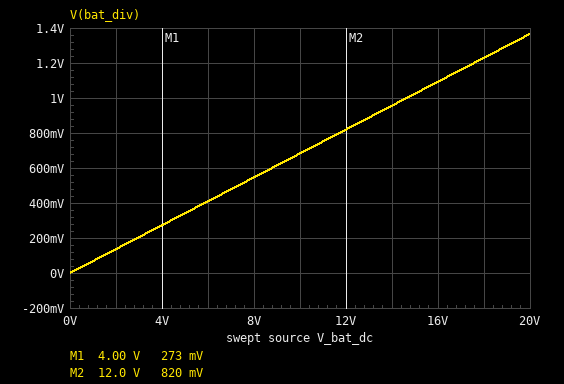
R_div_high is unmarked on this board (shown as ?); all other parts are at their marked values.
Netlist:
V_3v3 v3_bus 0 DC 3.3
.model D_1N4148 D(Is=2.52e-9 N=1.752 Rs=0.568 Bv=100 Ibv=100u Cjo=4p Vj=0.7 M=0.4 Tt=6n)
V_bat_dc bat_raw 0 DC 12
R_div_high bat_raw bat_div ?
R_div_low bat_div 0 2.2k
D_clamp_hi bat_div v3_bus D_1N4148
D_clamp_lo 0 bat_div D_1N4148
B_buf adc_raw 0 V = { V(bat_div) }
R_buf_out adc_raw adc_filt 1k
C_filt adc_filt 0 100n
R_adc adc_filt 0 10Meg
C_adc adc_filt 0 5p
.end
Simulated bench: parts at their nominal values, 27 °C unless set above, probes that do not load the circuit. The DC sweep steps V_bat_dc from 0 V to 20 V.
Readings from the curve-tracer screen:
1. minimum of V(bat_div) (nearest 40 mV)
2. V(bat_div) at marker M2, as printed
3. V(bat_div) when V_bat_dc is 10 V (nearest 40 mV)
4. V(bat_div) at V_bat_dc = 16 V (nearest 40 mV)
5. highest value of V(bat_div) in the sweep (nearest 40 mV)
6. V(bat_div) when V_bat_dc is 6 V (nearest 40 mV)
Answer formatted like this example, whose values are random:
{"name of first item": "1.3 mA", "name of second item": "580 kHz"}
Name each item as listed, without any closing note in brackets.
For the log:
{"minimum of V(bat_div)": "0 V", "V(bat_div) at marker M2, as printed": "820 mV", "V(bat_div) when V_bat_dc is 10 V": "680 mV", "V(bat_div) at V_bat_dc = 16 V": "1.08 V", "highest value of V(bat_div) in the sweep": "1.36 V", "V(bat_div) when V_bat_dc is 6 V": "400 mV"}
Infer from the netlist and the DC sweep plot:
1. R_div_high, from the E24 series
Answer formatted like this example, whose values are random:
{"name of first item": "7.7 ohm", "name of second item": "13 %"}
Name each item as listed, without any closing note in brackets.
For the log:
{"R_div_high, from the E24 series": "30 kΩ"}
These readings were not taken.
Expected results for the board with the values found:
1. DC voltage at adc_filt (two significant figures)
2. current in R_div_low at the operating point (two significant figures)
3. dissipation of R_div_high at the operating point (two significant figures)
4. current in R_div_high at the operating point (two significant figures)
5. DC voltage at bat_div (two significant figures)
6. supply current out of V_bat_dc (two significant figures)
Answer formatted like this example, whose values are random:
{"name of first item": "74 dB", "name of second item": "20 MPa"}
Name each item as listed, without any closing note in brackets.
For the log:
{"DC voltage at adc_filt": "820 mV", "current in R_div_low at the operating point": "370 µA", "dissipation of R_div_high at the operating point": "4.2 mW", "current in R_div_high at the operating point": "370 µA", "DC voltage at bat_div": "820 mV", "supply current out of V_bat_dc": "370 µA"}
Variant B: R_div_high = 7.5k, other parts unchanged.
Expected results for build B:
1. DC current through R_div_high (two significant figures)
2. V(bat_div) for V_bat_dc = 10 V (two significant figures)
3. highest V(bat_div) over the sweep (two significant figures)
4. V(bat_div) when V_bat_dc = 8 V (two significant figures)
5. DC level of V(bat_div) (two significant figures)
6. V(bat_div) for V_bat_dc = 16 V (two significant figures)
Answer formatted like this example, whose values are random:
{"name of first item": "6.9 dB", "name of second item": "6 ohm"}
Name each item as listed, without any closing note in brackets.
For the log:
{"DC current through R_div_high": "1.2 mA", "V(bat_div) for V_bat_dc = 10 V": "2.3 V", "highest V(bat_div) over the sweep": "3.8 V", "V(bat_div) when V_bat_dc = 8 V": "1.8 V", "DC level of V(bat_div)": "2.7 V", "V(bat_div) for V_bat_dc = 16 V": "3.6 V"}
